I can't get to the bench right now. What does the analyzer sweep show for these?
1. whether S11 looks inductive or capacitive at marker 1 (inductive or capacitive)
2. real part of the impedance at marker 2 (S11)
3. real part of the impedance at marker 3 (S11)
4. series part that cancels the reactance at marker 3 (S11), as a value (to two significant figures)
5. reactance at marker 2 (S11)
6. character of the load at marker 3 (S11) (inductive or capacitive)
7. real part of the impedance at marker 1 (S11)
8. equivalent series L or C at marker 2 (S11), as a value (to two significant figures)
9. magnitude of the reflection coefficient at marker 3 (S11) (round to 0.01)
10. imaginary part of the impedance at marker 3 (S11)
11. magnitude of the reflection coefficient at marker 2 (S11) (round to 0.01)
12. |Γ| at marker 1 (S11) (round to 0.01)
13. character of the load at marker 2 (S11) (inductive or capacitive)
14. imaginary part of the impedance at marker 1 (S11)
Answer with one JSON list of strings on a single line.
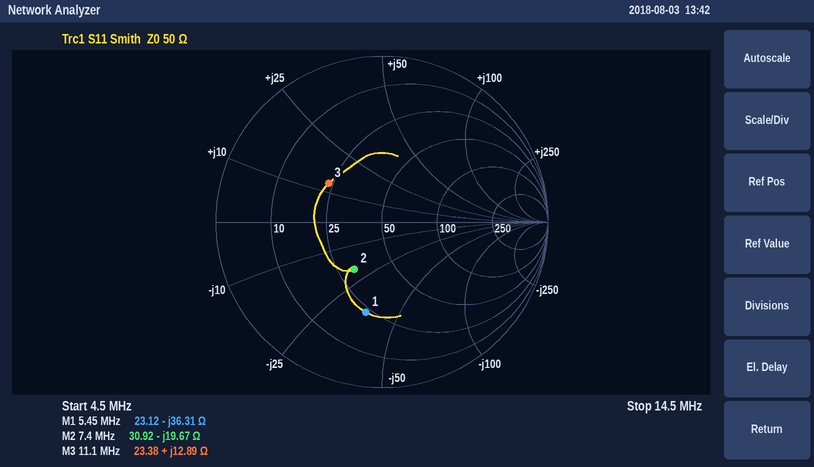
["capacitive", "30.92 Ω", "23.38 Ω", "1.1 nF", "-19.67 Ω", "inductive", "23.12 Ω", "1.1 nF", "0.40", "+12.89 Ω", "0.33", "0.55", "capacitive", "-36.31 Ω"]
